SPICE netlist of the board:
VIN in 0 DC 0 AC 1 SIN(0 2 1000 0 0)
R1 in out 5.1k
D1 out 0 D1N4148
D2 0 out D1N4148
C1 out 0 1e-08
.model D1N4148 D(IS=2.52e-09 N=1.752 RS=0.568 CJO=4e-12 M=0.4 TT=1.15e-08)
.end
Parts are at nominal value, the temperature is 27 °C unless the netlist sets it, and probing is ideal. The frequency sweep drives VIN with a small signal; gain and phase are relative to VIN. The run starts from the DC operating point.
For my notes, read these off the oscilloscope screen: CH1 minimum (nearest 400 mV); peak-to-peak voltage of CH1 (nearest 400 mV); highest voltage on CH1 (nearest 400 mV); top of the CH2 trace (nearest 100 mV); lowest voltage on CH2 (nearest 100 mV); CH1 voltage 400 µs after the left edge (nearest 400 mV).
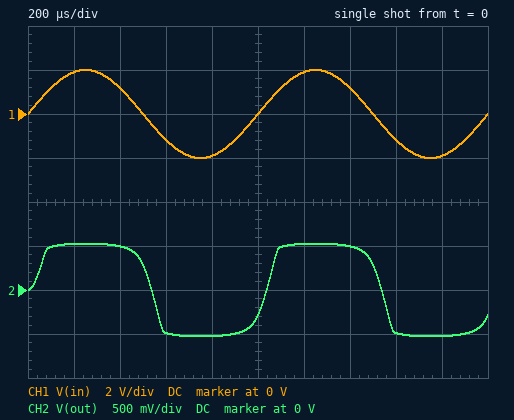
-2.0 V
4.0 V
2.0 V
500 mV
-500 mV
1.2 V
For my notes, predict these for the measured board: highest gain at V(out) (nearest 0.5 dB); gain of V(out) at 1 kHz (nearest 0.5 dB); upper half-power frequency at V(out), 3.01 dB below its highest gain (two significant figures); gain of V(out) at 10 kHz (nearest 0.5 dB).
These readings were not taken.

0 dB
-0.5 dB
3.1 kHz
-10.5 dB
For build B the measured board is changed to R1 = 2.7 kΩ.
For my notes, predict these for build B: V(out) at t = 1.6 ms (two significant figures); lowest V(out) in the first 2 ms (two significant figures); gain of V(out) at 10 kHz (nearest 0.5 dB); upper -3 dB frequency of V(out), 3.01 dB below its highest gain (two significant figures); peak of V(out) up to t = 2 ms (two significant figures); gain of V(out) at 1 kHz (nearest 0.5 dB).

-520 mV
-560 mV
-6.0 dB
5.9 kHz
560 mV
0 dB
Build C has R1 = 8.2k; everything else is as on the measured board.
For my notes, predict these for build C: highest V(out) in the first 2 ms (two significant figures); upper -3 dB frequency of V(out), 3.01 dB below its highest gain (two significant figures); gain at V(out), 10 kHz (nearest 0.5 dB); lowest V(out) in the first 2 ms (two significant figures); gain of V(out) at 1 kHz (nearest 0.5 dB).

510 mV
1.9 kHz
-14.5 dB
-510 mV
-1.0 dB
